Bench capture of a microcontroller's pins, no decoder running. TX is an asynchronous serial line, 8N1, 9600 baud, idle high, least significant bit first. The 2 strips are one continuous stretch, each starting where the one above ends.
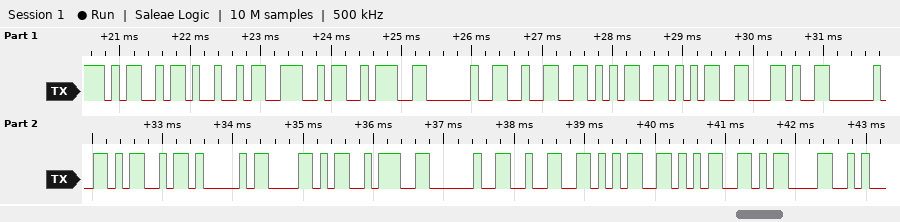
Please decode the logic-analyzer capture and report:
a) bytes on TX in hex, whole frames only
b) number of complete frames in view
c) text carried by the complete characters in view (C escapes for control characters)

4D 49 4E 3A 20 32 35 35 2C 20 4D 41 58 3A 20 32 35 35 0D
19
"MIN: 255, MAX: 255\r"
